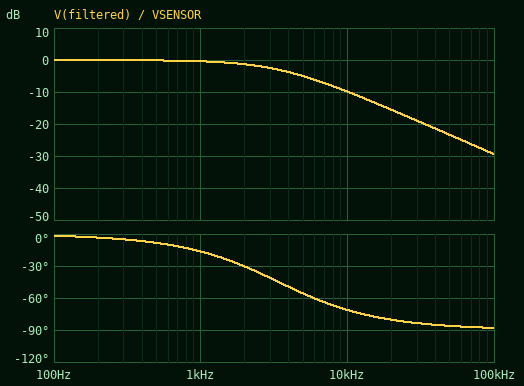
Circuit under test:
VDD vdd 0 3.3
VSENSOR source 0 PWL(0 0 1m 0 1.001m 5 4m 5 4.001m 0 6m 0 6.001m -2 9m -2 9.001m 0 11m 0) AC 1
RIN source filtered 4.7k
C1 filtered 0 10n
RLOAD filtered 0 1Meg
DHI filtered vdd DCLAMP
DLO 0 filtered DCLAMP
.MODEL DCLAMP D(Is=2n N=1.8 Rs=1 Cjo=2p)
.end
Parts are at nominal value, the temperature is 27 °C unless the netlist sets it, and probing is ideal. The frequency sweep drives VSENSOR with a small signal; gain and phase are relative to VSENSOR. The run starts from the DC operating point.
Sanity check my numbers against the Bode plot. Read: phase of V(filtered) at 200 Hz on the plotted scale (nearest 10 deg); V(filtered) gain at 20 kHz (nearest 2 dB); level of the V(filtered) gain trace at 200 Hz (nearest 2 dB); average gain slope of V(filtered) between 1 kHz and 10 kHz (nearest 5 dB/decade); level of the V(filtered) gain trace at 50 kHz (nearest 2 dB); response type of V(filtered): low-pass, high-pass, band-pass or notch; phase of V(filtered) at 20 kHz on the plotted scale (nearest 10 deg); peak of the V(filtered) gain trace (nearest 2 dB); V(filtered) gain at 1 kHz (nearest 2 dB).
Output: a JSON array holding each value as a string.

["0 deg", "-16 dB", "0 dB", "-10 dB/decade", "-24 dB", "low-pass", "-80 deg", "0 dB", "0 dB"]
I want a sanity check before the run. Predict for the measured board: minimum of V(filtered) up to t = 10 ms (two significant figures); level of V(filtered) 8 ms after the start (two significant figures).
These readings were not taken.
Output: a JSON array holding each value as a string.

["-560 mV", "-560 mV"]
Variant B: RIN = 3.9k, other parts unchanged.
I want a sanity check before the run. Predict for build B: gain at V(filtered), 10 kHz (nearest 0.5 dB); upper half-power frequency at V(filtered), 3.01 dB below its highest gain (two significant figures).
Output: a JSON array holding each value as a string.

["-8.5 dB", "4.1 kHz"]
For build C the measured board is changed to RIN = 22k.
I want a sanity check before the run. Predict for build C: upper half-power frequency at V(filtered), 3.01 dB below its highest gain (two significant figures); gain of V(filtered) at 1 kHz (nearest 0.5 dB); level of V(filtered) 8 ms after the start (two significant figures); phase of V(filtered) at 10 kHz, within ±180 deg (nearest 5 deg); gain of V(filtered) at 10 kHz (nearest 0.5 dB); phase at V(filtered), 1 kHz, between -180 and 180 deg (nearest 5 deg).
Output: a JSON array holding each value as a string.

["740 Hz", "-4.5 dB", "-490 mV", "-85 deg", "-23.0 dB", "-55 deg"]
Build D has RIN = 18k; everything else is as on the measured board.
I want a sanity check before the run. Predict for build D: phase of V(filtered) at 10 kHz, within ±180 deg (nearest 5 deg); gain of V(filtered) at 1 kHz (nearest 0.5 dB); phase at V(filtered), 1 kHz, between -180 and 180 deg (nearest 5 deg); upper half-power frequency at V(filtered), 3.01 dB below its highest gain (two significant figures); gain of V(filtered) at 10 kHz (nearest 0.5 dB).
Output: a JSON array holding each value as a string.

["-85 deg", "-3.5 dB", "-50 deg", "900 Hz", "-21.0 dB"]
